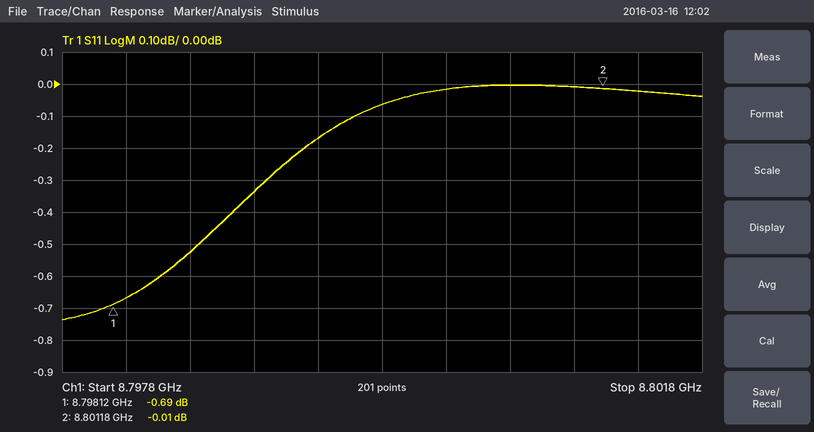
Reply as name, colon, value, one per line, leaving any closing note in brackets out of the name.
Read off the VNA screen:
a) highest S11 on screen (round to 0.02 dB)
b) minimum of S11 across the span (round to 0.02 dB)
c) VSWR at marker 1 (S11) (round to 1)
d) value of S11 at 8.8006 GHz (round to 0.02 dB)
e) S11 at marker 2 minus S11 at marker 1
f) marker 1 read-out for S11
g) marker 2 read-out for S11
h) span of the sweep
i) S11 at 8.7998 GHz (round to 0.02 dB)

highest S11 on screen: 0.00 dB
minimum of S11 across the span: -0.74 dB
VSWR at marker 1 (S11): 25
value of S11 at 8.8006 GHz: 0.00 dB
S11 at marker 2 minus S11 at marker 1: 0.68 dB
marker 1 read-out for S11: -0.69 dB
marker 2 read-out for S11: -0.01 dB
span of the sweep: 4 MHz
S11 at 8.7998 GHz: -0.06 dB
